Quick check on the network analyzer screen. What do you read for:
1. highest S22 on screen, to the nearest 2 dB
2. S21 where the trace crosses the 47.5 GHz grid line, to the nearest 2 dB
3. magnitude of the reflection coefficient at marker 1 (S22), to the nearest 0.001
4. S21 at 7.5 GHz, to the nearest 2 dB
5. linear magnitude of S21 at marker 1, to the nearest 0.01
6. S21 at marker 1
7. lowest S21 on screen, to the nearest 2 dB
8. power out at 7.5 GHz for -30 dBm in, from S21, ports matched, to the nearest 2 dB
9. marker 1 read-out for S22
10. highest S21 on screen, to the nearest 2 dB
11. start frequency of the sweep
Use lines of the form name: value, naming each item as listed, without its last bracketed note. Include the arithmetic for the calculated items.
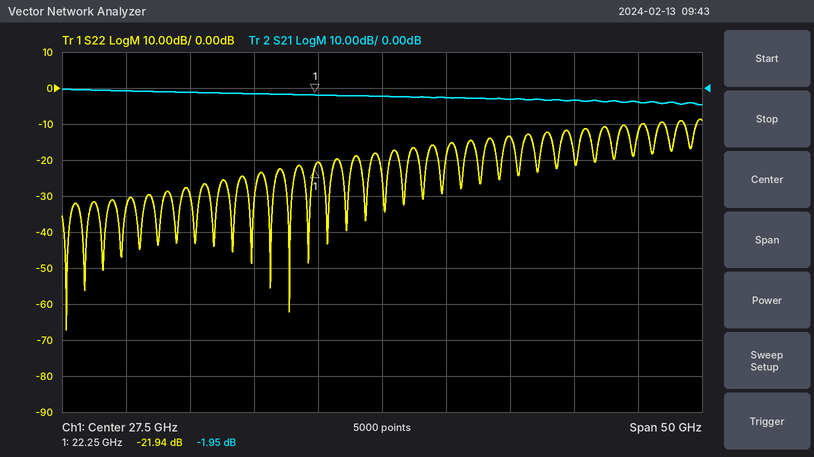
highest S22 on screen, to the nearest 2 dB: -8 dB
S21 where the trace crosses the 47.5 GHz grid line, to the nearest 2 dB: -4 dB
magnitude of the reflection coefficient at marker 1 (S22), to the nearest 0.001: 10^(-21.94/20) ≈ 0.080
S21 at 7.5 GHz, to the nearest 2 dB: 0 dB
linear magnitude of S21 at marker 1, to the nearest 0.01: 10^(-1.95/20) ≈ 0.80
S21 at marker 1: -1.95 dB
lowest S21 on screen, to the nearest 2 dB: -4 dB
power out at 7.5 GHz for -30 dBm in, from S21, ports matched, to the nearest 2 dB: -30 dBm + (0 dB) = -30 dBm
marker 1 read-out for S22: -21.94 dB
highest S21 on screen, to the nearest 2 dB: 0 dB
start frequency of the sweep: 2.5 GHz
